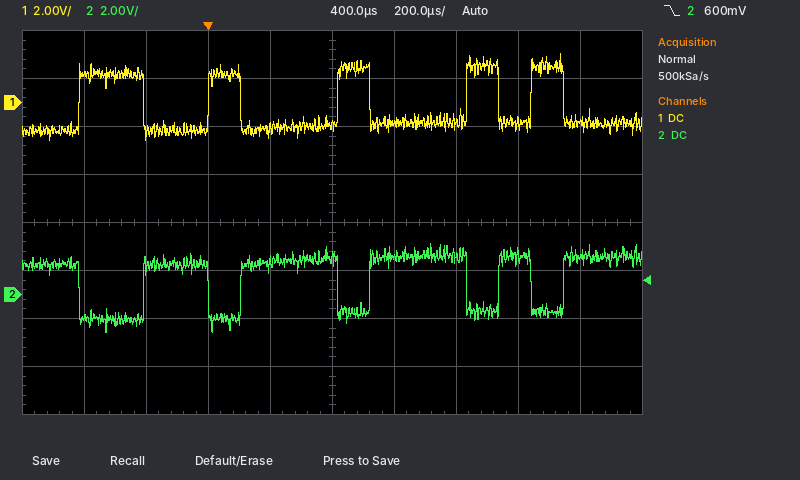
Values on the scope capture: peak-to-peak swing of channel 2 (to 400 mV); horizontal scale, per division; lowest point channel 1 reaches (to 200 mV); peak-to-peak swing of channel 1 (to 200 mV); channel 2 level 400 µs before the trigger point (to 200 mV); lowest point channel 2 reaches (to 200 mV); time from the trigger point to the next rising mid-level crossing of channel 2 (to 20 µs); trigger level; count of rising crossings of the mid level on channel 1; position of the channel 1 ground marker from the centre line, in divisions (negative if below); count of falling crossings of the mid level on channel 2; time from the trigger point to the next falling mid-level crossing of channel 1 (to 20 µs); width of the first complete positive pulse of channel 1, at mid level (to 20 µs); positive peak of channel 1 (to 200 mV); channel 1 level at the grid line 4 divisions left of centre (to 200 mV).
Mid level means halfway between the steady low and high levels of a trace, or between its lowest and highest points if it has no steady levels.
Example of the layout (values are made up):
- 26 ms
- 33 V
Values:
- 3.6 V
- 200 µs
- -1.6 V
- 3.6 V
- -1.0 V
- -1.6 V
- 100 µs
- 600 mV
- 5
- +2.5 div
- 5
- 100 µs
- 200 µs
- 2.0 V
- 1.2 V
